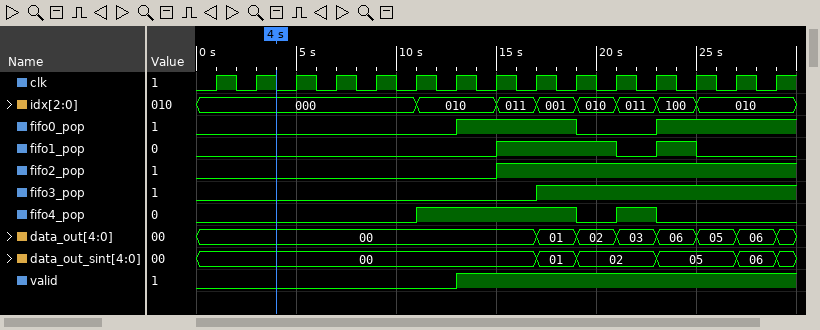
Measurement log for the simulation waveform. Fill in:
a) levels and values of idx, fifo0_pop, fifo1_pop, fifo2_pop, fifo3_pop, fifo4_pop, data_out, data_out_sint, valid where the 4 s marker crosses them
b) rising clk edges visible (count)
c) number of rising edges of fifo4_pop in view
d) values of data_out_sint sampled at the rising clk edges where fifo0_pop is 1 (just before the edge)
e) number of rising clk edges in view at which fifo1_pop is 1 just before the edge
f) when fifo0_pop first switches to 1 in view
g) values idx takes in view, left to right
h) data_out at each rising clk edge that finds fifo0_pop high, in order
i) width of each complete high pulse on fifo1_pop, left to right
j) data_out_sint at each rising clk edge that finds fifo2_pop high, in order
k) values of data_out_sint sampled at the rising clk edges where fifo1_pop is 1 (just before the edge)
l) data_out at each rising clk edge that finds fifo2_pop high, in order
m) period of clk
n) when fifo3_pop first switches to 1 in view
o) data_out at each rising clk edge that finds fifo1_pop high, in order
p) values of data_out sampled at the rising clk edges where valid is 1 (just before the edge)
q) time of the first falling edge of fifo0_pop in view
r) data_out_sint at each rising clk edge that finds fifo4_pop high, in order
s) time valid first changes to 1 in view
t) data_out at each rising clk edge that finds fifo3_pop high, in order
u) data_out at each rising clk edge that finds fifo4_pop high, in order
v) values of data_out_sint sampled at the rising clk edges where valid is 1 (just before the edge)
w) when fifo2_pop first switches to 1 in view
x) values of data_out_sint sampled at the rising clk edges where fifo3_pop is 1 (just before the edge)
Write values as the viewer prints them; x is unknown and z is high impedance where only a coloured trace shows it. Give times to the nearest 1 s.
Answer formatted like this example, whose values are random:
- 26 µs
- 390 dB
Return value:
- idx=000, fifo0_pop=0, fifo1_pop=0, fifo2_pop=0, fifo3_pop=0, fifo4_pop=0, data_out=00, data_out_sint=00, valid=0
- 15
- 2
- 00, 00, 01, 05, 05, 06
- 4
- 13 s
- 000, 010, 011, 001, 010, 011, 100, 010
- 00, 00, 01, 06, 05, 06
- 6 s, 2 s
- 00, 01, 02, 02, 05, 05, 06
- 00, 01, 02, 05
- 00, 01, 02, 03, 06, 05, 06
- 2 s
- 17 s
- 00, 01, 02, 06
- 00, 00, 01, 02, 03, 06, 05, 06
- 19 s
- 00, 00, 00, 01, 02
- 13 s
- 01, 02, 03, 06, 05, 06
- 00, 00, 00, 01, 03
- 00, 00, 01, 02, 02, 05, 05, 06
- 15 s
- 01, 02, 02, 05, 05, 06
